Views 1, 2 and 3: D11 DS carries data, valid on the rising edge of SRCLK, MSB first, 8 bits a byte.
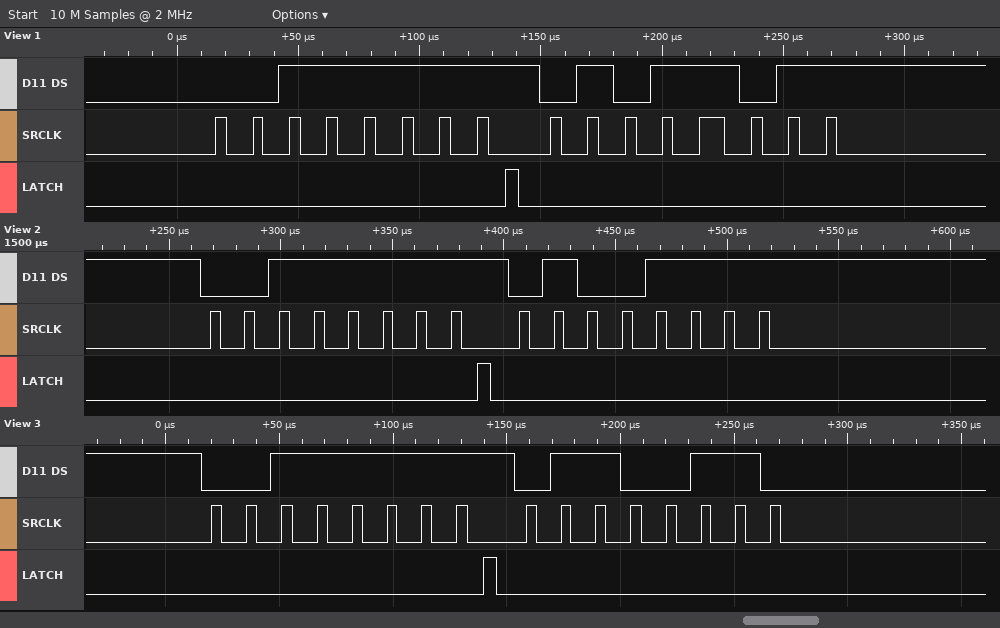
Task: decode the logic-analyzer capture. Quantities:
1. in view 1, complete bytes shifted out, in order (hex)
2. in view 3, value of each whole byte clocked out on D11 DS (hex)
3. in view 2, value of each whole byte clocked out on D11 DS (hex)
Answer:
3F 5B
3F 66
3F 4F
